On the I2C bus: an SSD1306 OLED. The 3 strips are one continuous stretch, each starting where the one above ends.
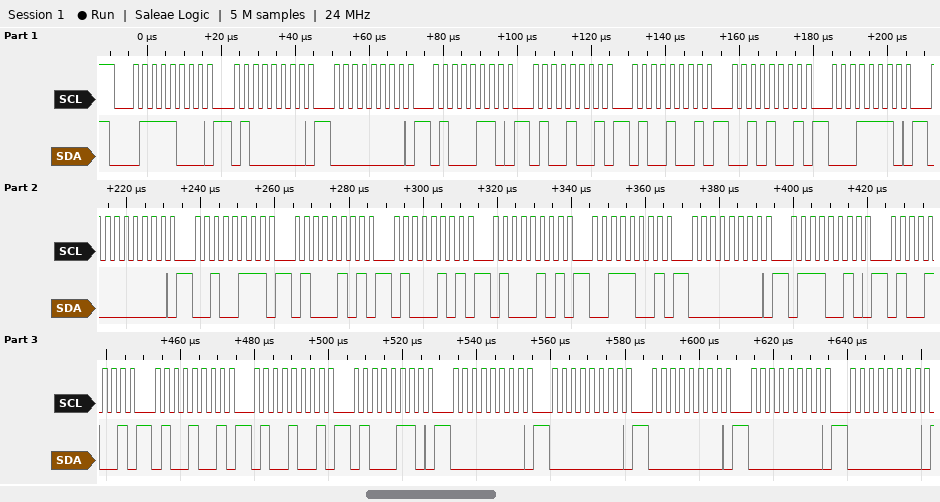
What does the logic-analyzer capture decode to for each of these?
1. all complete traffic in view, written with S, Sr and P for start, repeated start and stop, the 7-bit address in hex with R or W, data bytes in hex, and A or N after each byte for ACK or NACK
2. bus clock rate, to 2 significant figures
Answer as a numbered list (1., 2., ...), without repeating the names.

1. S 3CW A 40 A 00 A 46 A 49 A 49 A 29 A 1E A 00 A 27 A 45 A 45 A 45 A 39 A 00 A 72 A 49 A 49 A 49 A 46 A 00 A 00 A 00 A 00 A 00 A
2. 400 kHz
